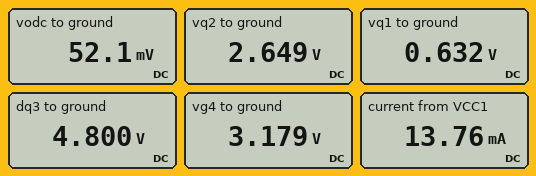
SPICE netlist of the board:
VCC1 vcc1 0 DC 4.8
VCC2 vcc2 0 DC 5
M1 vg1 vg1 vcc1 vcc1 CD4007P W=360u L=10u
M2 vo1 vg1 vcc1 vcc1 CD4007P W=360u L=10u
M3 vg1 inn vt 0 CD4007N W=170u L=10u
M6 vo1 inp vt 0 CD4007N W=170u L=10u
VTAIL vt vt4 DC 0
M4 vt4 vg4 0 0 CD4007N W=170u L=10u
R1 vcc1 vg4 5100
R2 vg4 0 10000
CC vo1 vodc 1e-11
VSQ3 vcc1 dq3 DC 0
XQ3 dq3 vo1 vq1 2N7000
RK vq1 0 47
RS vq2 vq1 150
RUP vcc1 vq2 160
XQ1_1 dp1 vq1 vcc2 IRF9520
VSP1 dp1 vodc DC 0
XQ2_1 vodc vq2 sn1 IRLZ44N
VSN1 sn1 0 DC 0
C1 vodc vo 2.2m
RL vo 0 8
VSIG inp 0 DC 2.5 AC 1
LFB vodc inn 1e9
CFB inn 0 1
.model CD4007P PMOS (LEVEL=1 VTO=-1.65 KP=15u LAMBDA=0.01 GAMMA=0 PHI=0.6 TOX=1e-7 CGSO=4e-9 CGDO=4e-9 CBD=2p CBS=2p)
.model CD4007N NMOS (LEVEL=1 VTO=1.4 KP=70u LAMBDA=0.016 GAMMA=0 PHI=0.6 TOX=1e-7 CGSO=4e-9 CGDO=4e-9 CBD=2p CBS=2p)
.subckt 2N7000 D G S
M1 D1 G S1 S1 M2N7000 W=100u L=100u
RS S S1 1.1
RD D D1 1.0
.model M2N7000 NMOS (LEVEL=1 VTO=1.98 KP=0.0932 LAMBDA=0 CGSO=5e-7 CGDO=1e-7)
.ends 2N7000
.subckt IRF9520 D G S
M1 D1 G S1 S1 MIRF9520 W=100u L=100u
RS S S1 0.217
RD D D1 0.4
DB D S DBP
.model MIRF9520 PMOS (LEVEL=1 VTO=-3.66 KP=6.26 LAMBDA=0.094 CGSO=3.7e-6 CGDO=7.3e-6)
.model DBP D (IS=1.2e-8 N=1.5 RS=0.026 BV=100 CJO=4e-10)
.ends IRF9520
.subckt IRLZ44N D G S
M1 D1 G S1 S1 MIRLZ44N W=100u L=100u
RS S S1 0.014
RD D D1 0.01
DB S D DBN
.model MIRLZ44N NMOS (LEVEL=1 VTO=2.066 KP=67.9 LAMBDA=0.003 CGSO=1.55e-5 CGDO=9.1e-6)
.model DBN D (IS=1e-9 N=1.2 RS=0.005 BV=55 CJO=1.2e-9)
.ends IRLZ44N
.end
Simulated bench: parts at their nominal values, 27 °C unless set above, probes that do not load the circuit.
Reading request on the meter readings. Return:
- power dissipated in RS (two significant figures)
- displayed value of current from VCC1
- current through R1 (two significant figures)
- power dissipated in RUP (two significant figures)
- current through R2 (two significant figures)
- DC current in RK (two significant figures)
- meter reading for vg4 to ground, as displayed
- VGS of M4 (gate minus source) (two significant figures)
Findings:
27 mW
13.76 mA
320 µA
29 mW
320 µA
13 mA
3.179 V
3.2 V
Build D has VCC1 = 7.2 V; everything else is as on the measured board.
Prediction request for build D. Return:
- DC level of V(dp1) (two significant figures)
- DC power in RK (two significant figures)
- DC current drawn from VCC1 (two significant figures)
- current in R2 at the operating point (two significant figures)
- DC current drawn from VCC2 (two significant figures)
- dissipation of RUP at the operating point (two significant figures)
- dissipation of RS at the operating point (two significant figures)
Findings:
13 mV
19 mW
21 mA
480 µA
410 mA
65 mW
61 mW
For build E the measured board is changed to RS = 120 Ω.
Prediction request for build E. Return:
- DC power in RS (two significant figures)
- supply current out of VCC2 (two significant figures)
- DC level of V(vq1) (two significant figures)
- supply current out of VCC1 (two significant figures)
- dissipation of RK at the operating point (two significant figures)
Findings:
26 mW
910 mA
690 mV
15 mA
10 mW
